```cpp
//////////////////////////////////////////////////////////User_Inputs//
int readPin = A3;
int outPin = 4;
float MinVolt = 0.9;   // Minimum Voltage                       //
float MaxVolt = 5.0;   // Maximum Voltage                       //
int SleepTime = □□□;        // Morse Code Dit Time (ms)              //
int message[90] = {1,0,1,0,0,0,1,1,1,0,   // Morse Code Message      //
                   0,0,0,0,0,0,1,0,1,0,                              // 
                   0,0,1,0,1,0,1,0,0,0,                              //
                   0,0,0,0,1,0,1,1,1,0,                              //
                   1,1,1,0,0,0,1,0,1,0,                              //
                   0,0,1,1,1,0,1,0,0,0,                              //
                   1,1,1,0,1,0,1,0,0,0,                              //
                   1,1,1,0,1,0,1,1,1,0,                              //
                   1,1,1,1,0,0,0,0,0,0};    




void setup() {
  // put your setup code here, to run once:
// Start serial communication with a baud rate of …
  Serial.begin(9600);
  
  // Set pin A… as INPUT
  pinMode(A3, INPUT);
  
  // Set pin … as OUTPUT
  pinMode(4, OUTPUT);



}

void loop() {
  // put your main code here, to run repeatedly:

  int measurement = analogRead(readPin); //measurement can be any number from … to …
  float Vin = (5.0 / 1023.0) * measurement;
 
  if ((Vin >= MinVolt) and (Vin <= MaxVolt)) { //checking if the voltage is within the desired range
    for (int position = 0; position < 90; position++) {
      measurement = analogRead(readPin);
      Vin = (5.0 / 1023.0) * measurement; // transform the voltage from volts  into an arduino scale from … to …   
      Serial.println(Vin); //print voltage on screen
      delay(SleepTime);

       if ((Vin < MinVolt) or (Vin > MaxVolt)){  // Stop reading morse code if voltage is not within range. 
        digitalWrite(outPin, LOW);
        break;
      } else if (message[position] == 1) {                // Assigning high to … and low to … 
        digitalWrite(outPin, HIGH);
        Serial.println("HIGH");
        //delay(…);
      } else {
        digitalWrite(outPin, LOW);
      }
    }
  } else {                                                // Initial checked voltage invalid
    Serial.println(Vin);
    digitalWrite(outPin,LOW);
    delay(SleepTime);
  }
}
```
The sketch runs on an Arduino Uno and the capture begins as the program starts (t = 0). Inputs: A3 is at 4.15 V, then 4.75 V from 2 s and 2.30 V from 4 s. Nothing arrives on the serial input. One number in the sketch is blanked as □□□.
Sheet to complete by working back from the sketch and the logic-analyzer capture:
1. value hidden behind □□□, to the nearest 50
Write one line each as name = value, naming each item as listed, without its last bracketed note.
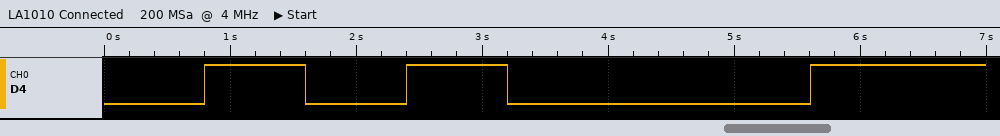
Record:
value hidden behind □□□, to the nearest 50 = 800
